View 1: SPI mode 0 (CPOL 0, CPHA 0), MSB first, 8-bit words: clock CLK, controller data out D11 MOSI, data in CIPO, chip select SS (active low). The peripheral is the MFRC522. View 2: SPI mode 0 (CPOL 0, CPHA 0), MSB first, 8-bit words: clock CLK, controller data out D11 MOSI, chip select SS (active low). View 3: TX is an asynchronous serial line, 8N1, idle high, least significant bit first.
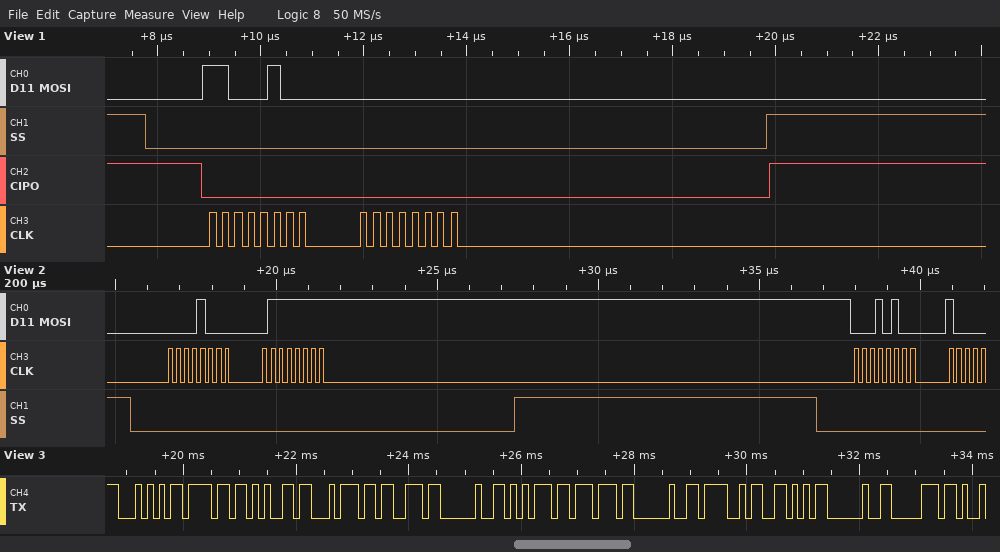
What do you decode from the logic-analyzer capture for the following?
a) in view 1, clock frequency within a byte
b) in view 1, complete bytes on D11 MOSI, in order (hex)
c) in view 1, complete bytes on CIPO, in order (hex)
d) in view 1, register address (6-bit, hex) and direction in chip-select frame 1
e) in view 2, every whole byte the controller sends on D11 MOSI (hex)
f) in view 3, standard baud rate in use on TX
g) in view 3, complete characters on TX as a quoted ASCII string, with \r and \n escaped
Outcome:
4 MHz
0xC4 0x00
0x00 0x00
0x22 read
0x08 0x7F 0x14
9600 baud
"Toets uw OV p"
